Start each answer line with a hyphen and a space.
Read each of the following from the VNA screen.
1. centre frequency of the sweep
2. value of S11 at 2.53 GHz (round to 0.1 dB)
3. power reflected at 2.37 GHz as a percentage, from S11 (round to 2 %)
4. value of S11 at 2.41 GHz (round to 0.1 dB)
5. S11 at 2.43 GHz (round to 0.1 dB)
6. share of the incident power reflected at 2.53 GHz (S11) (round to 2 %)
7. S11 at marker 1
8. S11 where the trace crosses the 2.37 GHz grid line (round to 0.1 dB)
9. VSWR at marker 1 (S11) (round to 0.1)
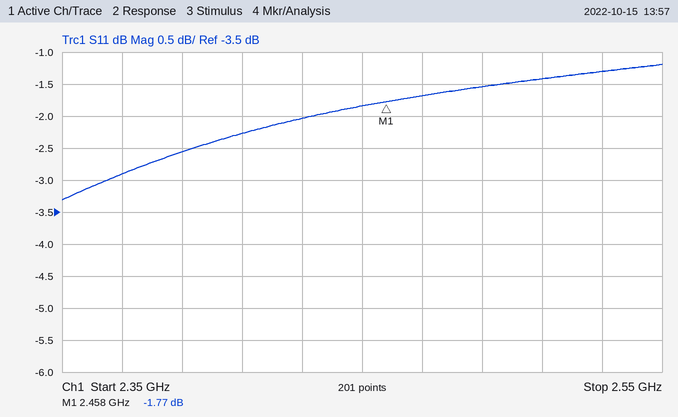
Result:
- 2.45 GHz
- -1.3 dB
- 52 %
- -2.3 dB
- -2.0 dB
- 74 %
- -1.77 dB
- -2.9 dB
- 9.8
